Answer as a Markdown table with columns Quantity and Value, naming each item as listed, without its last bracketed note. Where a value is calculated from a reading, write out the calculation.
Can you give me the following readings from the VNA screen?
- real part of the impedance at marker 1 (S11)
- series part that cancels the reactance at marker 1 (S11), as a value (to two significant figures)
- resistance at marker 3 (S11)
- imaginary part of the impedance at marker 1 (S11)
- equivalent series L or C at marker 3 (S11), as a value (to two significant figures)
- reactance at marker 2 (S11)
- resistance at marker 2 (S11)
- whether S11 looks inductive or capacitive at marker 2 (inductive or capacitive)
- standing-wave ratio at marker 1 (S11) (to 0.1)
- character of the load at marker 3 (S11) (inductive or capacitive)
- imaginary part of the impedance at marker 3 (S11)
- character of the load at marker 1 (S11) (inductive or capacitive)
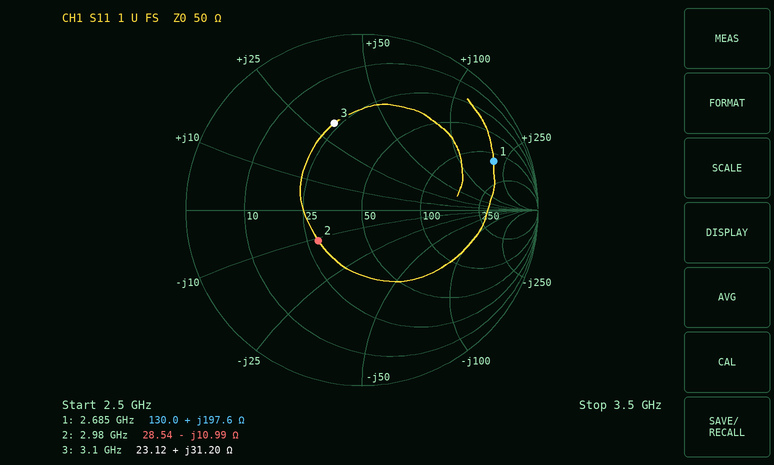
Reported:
| Quantity | Value |
|---|---|
| real part of the impedance at marker 1 | 130.0 Ω |
| series part that cancels the reactance at marker 1 (S11), as a value | C = 1/(2π × 2.685 GHz × 197.6 Ω) ≈ 300 fF |
| resistance at marker 3 | 23.12 Ω |
| imaginary part of the impedance at marker 1 | +197.6 Ω |
| equivalent series L or C at marker 3 (S11), as a value | L = 31.2 Ω/(2π × 3.1 GHz) ≈ 1.6 nH |
| reactance at marker 2 | -10.99 Ω |
| resistance at marker 2 | 28.54 Ω |
| whether S11 looks inductive or capacitive at marker 2 | capacitive |
| standing-wave ratio at marker 1 (S11) | 8.9 |
| character of the load at marker 3 (S11) | inductive |
| imaginary part of the impedance at marker 3 | +31.20 Ω |
| character of the load at marker 1 (S11) | inductive |
